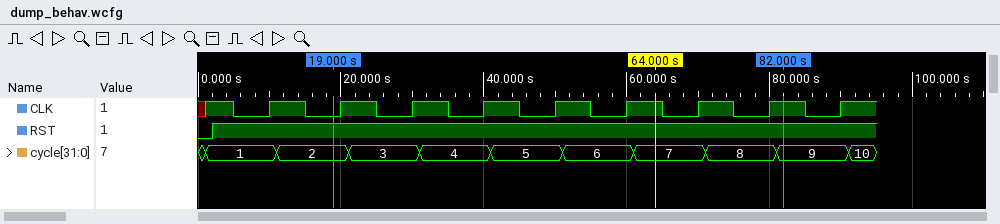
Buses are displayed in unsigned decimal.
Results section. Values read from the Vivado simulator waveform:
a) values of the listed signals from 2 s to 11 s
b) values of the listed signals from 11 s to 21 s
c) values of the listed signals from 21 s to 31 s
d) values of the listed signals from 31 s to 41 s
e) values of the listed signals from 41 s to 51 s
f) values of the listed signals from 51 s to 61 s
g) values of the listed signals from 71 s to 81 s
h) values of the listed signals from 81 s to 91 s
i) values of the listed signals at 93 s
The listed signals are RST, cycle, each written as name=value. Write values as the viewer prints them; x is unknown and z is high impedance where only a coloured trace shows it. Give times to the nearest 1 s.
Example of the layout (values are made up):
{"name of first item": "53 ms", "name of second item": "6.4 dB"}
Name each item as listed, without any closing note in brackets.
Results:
{"values of the listed signals from 2 s to 11 s": "RST=1, cycle=1", "values of the listed signals from 11 s to 21 s": "RST=1, cycle=2", "values of the listed signals from 21 s to 31 s": "RST=1, cycle=3", "values of the listed signals from 31 s to 41 s": "RST=1, cycle=4", "values of the listed signals from 41 s to 51 s": "RST=1, cycle=5", "values of the listed signals from 51 s to 61 s": "RST=1, cycle=6", "values of the listed signals from 71 s to 81 s": "RST=1, cycle=8", "values of the listed signals from 81 s to 91 s": "RST=1, cycle=9", "values of the listed signals at 93 s": "RST=1, cycle=10"}
